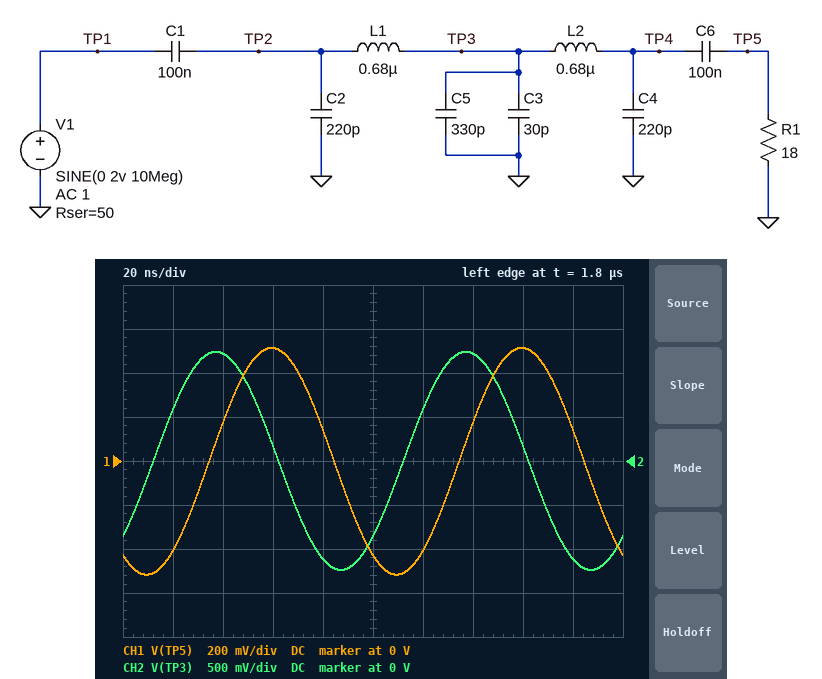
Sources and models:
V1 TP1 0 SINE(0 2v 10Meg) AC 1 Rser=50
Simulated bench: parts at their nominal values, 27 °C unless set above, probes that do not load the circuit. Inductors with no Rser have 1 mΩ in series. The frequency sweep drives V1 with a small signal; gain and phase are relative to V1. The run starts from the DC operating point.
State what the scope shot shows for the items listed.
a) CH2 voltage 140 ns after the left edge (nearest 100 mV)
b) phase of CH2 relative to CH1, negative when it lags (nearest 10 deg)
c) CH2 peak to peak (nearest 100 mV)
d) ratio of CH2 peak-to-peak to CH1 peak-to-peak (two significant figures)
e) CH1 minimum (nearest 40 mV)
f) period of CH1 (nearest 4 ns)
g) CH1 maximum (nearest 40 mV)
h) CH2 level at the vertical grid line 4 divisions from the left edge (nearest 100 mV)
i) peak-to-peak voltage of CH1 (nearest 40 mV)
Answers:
1.2 V
80 deg
2.5 V
2.4
-520 mV
100 ns
520 mV
-1.1 V
1.04 V
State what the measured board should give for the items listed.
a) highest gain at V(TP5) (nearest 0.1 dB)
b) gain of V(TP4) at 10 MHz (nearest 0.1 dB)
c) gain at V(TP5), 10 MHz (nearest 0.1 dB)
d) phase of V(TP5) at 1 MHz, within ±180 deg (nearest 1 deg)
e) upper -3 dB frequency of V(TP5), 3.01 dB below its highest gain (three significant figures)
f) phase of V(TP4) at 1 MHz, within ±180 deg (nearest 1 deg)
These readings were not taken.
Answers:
-11.1 dB
-11.8 dB
-11.8 dB
-8 deg
17.8 MHz
-13 deg
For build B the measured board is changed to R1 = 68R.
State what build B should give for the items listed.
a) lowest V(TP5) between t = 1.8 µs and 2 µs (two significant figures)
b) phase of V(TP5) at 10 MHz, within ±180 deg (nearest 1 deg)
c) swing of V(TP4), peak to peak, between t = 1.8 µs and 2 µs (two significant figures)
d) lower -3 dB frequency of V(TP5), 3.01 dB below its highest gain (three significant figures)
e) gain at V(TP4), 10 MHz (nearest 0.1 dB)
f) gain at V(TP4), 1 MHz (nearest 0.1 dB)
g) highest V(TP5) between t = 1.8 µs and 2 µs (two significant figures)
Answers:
-1.2 V
-125 deg
2.3 V
27.6 kHz
-4.7 dB
-4.8 dB
1.2 V
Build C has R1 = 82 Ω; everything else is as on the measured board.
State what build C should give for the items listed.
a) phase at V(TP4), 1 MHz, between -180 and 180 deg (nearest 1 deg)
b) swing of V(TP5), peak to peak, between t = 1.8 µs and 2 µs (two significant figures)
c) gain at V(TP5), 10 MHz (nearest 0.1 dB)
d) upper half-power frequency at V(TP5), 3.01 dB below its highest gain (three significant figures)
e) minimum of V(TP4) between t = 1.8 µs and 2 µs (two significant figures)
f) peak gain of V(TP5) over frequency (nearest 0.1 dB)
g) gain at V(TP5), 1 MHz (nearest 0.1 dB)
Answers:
-12 deg
2.5 V
-4.0 dB
19.3 MHz
-1.3 V
-3.9 dB
-4.2 dB
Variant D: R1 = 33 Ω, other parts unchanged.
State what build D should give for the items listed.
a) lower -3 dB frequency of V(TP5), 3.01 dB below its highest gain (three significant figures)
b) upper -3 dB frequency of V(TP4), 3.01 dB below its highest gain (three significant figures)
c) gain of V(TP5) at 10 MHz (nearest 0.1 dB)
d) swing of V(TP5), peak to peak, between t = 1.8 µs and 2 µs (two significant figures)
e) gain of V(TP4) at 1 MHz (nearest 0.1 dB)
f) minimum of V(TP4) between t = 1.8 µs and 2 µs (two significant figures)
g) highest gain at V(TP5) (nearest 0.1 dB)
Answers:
39.8 kHz
17.4 MHz
-8.1 dB
1.6 V
-8.0 dB
-780 mV
-7.9 dB
